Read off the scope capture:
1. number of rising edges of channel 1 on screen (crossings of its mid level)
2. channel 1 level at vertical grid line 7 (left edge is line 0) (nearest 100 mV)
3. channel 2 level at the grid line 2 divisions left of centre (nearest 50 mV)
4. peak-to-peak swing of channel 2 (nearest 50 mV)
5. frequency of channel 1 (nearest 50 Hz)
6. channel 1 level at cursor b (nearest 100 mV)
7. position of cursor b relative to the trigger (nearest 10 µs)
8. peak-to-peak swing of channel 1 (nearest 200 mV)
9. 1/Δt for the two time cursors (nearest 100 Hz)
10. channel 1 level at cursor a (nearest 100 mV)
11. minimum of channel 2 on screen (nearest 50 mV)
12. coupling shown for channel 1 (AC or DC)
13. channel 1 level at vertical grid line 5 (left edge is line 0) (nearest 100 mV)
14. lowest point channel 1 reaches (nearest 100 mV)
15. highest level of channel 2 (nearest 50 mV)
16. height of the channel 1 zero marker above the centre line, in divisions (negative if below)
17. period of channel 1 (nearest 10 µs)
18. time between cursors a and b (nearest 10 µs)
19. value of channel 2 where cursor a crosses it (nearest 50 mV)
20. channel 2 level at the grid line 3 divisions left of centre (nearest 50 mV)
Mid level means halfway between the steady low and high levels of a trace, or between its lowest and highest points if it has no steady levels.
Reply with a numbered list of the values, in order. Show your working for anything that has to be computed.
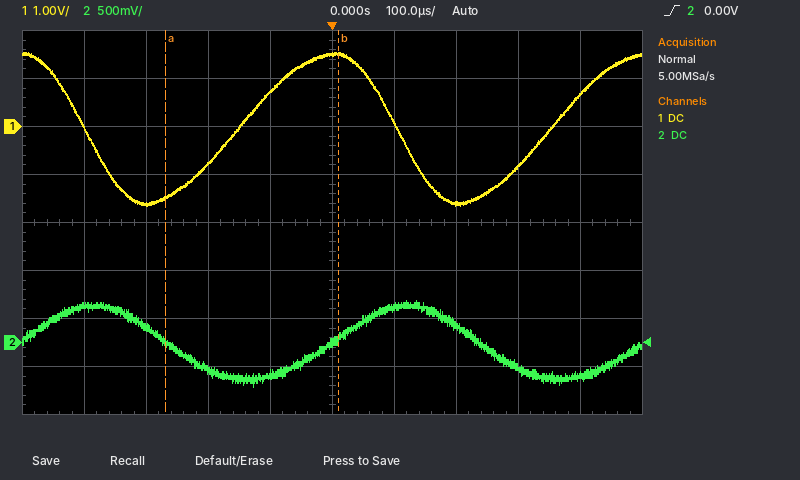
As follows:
1. 2
2. -1.6 V
3. -300 mV
4. 450 mV − (-450 mV) = 900 mV
5. 1 / 500 µs ≈ 2.00 kHz
6. 1.5 V
7. +10 µs
8. 3.2 V
9. 1 / 280 µs ≈ 3.6 kHz
10. -1.5 V
11. -450 mV
12. DC
13. 1.5 V
14. -1.6 V
15. 450 mV
16. +2.0 div
17. 500 µs
18. 280 µs
19. 0 mV
20. 150 mV
